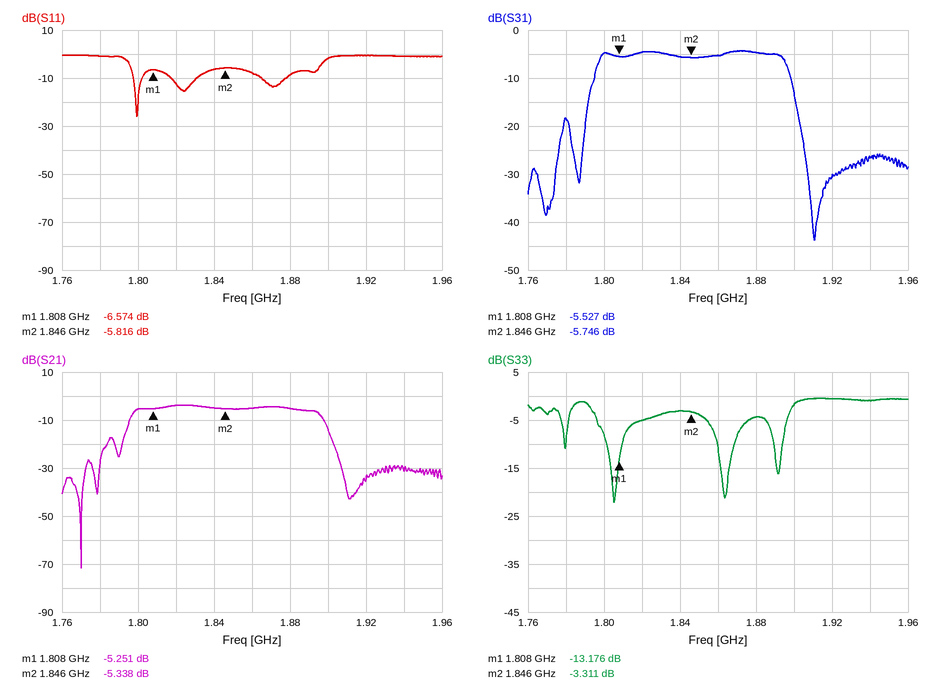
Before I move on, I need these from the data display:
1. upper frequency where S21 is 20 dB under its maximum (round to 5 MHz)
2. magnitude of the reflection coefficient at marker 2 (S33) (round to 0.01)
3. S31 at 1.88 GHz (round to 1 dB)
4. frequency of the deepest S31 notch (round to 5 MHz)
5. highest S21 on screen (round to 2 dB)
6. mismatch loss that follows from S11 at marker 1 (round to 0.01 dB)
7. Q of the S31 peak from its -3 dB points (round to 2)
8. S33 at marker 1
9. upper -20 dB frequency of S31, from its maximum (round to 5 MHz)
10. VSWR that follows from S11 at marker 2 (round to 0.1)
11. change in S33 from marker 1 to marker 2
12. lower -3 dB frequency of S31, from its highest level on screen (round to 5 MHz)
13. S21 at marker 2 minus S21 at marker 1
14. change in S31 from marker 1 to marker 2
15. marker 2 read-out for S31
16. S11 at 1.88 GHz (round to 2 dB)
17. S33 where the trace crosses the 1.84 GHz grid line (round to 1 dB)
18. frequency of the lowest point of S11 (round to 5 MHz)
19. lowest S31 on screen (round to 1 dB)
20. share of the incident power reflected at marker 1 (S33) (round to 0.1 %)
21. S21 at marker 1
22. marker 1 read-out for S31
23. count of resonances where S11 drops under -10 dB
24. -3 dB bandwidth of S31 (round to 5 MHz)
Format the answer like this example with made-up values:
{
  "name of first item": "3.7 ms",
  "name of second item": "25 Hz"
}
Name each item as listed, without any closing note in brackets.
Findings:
{
  "upper frequency where S21 is 20 dB under its maximum": "1.905 GHz",
  "magnitude of the reflection coefficient at marker 2 (S33)": "0.68",
  "S31 at 1.88 GHz": "-5 dB",
  "frequency of the deepest S31 notch": "1.910 GHz",
  "highest S21 on screen": "-4 dB",
  "mismatch loss that follows from S11 at marker 1": "1.08 dB",
  "Q of the S31 peak from its -3 dB points": "18",
  "S33 at marker 1": "-13.176 dB",
  "upper -20 dB frequency of S31, from its maximum": "1.905 GHz",
  "VSWR that follows from S11 at marker 2": "3.1",
  "change in S33 from marker 1 to marker 2": "9.865 dB",
  "lower -3 dB frequency of S31, from its highest level on screen": "1.795 GHz",
  "S21 at marker 2 minus S21 at marker 1": "-0.087 dB",
  "change in S31 from marker 1 to marker 2": "-0.219 dB",
  "marker 2 read-out for S31": "-5.746 dB",
  "S11 at 1.88 GHz": "-8 dB",
  "S33 where the trace crosses the 1.84 GHz grid line": "-3 dB",
  "frequency of the lowest point of S11": "1.800 GHz",
  "lowest S31 on screen": "-44 dB",
  "share of the incident power reflected at marker 1 (S33)": "4.8 %",
  "S21 at marker 1": "-5.251 dB",
  "marker 1 read-out for S31": "-5.527 dB",
  "count of resonances where S11 drops under -10 dB": "3",
  "-3 dB bandwidth of S31": "100 MHz"
}
